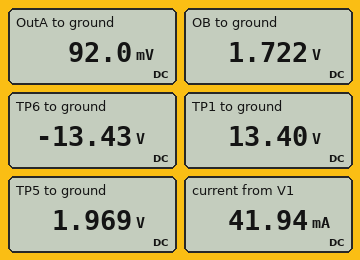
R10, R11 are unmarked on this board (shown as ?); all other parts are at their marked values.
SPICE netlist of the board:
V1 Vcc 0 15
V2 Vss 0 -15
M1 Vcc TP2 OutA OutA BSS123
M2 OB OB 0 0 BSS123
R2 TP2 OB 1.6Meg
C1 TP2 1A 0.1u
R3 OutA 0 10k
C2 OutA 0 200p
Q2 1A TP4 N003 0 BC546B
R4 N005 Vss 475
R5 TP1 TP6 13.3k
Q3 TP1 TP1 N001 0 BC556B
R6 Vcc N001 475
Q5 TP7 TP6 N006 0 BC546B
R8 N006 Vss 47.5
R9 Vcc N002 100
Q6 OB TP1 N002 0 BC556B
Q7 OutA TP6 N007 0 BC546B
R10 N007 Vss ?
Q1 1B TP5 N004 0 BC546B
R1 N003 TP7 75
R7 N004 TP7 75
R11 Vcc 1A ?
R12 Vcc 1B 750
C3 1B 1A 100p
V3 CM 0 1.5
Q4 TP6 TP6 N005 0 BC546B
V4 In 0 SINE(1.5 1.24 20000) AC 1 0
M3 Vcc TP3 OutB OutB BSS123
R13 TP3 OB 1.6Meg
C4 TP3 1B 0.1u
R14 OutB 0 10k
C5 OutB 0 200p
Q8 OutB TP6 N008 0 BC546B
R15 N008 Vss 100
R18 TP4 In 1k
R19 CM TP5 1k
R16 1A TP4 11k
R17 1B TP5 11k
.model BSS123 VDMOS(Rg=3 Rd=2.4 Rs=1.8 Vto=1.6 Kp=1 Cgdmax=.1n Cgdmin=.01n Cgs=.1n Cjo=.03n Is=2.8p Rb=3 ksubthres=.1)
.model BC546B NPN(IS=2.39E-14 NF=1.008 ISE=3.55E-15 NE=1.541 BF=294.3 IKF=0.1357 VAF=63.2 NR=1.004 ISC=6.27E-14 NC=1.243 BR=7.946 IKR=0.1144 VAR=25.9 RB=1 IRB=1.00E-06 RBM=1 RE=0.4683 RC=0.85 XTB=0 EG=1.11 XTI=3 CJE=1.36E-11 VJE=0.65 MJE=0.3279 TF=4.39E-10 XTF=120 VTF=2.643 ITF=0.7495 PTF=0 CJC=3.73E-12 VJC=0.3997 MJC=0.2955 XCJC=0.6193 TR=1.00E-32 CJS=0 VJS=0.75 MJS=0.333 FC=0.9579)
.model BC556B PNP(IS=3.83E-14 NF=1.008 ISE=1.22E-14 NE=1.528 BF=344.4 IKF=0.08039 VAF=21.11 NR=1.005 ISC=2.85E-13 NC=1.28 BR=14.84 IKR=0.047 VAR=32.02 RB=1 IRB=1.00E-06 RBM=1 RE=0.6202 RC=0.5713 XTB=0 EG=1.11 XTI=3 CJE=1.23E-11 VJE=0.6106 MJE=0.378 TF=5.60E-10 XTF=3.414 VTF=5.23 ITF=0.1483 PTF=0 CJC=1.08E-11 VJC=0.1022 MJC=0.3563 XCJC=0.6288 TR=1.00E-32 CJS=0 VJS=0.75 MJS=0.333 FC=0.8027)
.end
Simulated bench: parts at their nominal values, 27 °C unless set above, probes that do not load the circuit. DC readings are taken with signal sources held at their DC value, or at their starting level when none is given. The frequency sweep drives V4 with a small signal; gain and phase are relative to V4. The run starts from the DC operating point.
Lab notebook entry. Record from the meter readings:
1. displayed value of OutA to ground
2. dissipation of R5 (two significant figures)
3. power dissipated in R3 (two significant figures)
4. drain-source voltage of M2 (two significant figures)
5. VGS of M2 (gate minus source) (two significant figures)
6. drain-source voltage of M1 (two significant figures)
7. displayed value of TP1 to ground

92.0 mV
54 mW
850 nW
1.7 V
1.7 V
15 V
13.40 V
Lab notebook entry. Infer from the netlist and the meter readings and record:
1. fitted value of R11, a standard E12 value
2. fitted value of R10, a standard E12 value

1 kΩ
270 Ω
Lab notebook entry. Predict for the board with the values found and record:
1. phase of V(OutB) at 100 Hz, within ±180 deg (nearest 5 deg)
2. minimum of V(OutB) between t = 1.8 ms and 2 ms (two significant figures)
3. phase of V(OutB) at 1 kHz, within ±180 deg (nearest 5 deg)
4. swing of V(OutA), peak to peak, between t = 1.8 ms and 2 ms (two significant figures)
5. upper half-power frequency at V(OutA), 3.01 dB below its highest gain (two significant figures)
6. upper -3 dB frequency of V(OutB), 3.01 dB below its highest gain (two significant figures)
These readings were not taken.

0 deg
-2.7 V
0 deg
6.8 V
1.6 MHz
1.6 MHz
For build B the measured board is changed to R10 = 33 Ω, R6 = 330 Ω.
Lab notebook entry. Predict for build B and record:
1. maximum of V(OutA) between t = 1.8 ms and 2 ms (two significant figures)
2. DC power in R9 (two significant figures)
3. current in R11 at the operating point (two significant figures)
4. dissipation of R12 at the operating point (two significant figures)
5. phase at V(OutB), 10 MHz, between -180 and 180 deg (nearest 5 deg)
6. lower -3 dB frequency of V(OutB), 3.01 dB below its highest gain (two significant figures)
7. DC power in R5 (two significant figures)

3.2 V
4.2 mW
8.5 mA
72 mW
-130 deg
1.0 Hz
55 mW
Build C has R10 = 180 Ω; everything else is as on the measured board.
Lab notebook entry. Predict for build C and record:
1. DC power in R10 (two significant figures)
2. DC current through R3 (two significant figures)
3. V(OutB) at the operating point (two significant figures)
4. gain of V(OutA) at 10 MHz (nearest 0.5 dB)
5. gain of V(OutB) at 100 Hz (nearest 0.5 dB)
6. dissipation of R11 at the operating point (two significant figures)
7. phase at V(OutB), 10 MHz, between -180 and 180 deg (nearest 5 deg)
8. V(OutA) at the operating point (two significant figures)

4.4 mW
6.0 µA
5.1 mV
-10.0 dB
6.5 dB
75 mW
-120 deg
60 mV
